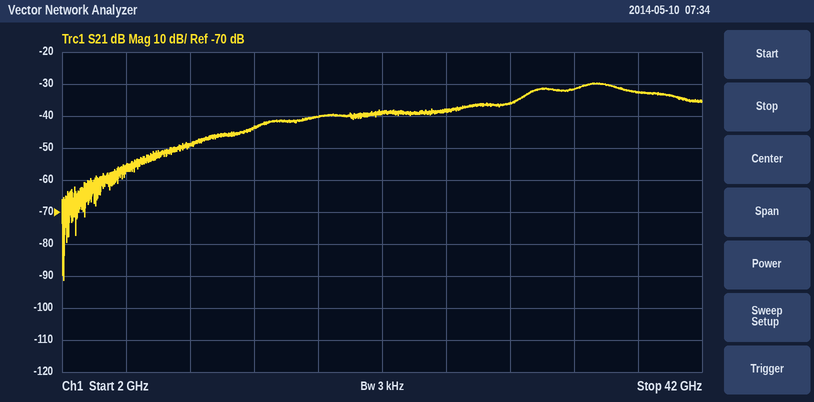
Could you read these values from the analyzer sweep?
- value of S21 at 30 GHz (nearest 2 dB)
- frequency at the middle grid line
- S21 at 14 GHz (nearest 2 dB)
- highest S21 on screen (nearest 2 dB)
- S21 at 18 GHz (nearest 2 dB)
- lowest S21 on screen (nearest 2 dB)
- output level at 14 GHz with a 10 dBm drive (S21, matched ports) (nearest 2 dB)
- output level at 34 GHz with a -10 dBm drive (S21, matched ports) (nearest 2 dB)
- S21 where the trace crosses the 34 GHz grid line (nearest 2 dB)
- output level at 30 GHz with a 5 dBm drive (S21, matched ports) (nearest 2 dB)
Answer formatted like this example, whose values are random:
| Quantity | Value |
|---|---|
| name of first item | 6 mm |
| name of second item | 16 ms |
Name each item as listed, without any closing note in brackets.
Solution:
| Quantity | Value |
|---|---|
| value of S21 at 30 GHz | -36 dB |
| frequency at the middle grid line | 22 GHz |
| S21 at 14 GHz | -44 dB |
| highest S21 on screen | -30 dB |
| S21 at 18 GHz | -40 dB |
| lowest S21 on screen | -92 dB |
| output level at 14 GHz with a 10 dBm drive (S21, matched ports) | -34 dBm |
| output level at 34 GHz with a -10 dBm drive (S21, matched ports) | -42 dBm |
| S21 where the trace crosses the 34 GHz grid line | -32 dB |
| output level at 30 GHz with a 5 dBm drive (S21, matched ports) | -32 dBm |
